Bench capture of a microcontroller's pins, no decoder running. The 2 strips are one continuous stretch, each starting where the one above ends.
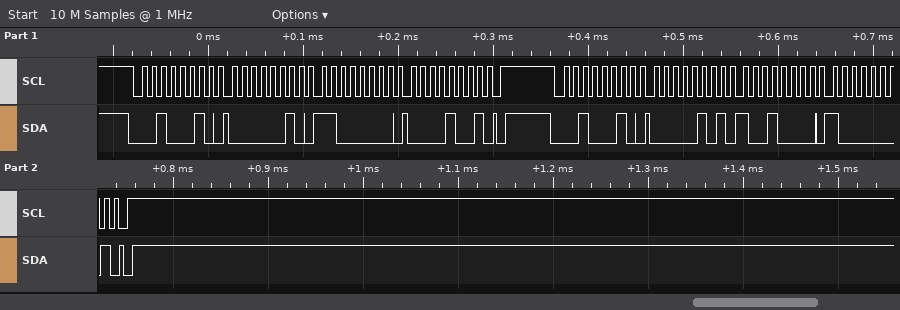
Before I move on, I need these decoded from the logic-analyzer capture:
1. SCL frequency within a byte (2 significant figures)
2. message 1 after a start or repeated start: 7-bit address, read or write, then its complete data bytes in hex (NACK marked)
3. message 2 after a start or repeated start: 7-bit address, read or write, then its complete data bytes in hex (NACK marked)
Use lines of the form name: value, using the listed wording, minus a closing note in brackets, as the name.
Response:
SCL frequency within a byte: 100 kHz
message 1 after a start or repeated start: 7-bit address, read or write, then its complete data bytes in hex: 0x11 write: 02 C0 09
message 2 after a start or repeated start: 7-bit address, read or write, then its complete data bytes in hex: 0x11 write: 05 90 81
